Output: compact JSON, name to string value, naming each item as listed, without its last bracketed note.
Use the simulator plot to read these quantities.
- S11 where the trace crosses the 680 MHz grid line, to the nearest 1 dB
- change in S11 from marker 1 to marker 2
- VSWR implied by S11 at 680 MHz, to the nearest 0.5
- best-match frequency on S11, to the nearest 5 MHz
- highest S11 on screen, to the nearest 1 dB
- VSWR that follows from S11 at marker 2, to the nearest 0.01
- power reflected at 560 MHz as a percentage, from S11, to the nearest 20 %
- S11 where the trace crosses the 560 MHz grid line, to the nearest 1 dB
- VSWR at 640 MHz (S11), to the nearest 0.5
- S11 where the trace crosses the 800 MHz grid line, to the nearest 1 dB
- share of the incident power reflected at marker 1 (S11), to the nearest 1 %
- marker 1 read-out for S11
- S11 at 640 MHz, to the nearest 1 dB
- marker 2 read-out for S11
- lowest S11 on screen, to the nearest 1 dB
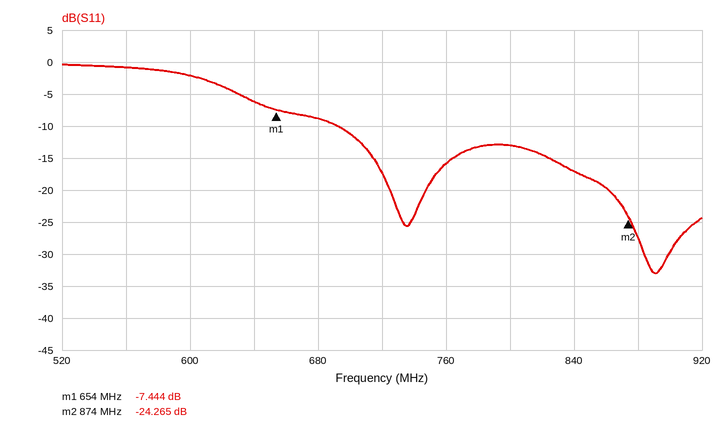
{"S11 where the trace crosses the 680 MHz grid line, to the nearest 1 dB": "-9 dB", "change in S11 from marker 1 to marker 2": "-16.821 dB", "VSWR implied by S11 at 680 MHz, to the nearest 0.5": "2.0", "best-match frequency on S11, to the nearest 5 MHz": "890 MHz", "highest S11 on screen, to the nearest 1 dB": "0 dB", "VSWR that follows from S11 at marker 2, to the nearest 0.01": "1.13", "power reflected at 560 MHz as a percentage, from S11, to the nearest 20 %": "80 %", "S11 where the trace crosses the 560 MHz grid line, to the nearest 1 dB": "-1 dB", "VSWR at 640 MHz (S11), to the nearest 0.5": "3.0", "S11 where the trace crosses the 800 MHz grid line, to the nearest 1 dB": "-13 dB", "share of the incident power reflected at marker 1 (S11), to the nearest 1 %": "18 %", "marker 1 read-out for S11": "-7.444 dB", "S11 at 640 MHz, to the nearest 1 dB": "-6 dB", "marker 2 read-out for S11": "-24.265 dB", "lowest S11 on screen, to the nearest 1 dB": "-33 dB"}
